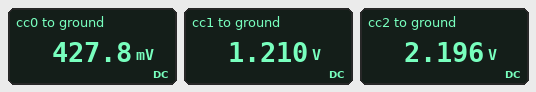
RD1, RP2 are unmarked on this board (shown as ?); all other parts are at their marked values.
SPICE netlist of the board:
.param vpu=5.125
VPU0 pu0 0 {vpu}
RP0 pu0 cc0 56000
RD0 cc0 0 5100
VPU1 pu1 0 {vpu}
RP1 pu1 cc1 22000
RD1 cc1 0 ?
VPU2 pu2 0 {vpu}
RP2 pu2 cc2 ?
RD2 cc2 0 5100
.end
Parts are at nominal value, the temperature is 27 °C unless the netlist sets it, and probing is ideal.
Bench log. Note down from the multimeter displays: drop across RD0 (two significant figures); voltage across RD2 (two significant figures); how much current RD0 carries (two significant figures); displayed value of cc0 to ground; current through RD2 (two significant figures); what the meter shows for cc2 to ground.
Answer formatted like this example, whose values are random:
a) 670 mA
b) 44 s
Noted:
a) 430 mV
b) 2.2 V
c) 84 µA
d) 427.8 mV
e) 430 µA
f) 2.196 V
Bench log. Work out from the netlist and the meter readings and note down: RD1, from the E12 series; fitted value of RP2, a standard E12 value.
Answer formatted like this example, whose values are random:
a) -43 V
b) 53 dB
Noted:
a) 6.8 kΩ
b) 6.8 kΩ
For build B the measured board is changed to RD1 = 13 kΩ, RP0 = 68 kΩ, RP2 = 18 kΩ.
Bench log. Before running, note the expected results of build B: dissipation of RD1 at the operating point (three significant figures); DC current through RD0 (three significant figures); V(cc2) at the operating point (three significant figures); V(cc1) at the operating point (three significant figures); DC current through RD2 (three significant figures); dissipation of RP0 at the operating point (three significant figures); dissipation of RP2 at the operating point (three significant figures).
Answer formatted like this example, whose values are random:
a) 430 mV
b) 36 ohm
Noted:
a) 279 µW
b) 70.1 µA
c) 1.13 V
d) 1.90 V
e) 222 µA
f) 334 µW
g) 886 µW
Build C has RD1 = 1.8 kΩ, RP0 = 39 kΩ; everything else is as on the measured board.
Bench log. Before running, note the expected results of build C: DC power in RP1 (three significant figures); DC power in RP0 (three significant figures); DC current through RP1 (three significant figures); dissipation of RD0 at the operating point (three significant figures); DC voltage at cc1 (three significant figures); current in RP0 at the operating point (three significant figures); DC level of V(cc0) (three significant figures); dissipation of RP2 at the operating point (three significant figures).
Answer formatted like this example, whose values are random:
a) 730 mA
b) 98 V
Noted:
a) 1.02 mW
b) 527 µW
c) 215 µA
d) 68.9 µW
e) 388 mV
f) 116 µA
g) 593 mV
h) 1.26 mW
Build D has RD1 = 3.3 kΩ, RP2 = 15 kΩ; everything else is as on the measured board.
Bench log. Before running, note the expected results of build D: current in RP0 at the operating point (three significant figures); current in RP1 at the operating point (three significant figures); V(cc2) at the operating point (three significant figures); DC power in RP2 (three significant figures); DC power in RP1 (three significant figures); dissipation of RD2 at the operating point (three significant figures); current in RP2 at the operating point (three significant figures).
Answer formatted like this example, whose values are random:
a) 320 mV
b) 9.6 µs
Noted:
a) 83.9 µA
b) 203 µA
c) 1.30 V
d) 975 µW
e) 903 µW
f) 332 µW
g) 255 µA
